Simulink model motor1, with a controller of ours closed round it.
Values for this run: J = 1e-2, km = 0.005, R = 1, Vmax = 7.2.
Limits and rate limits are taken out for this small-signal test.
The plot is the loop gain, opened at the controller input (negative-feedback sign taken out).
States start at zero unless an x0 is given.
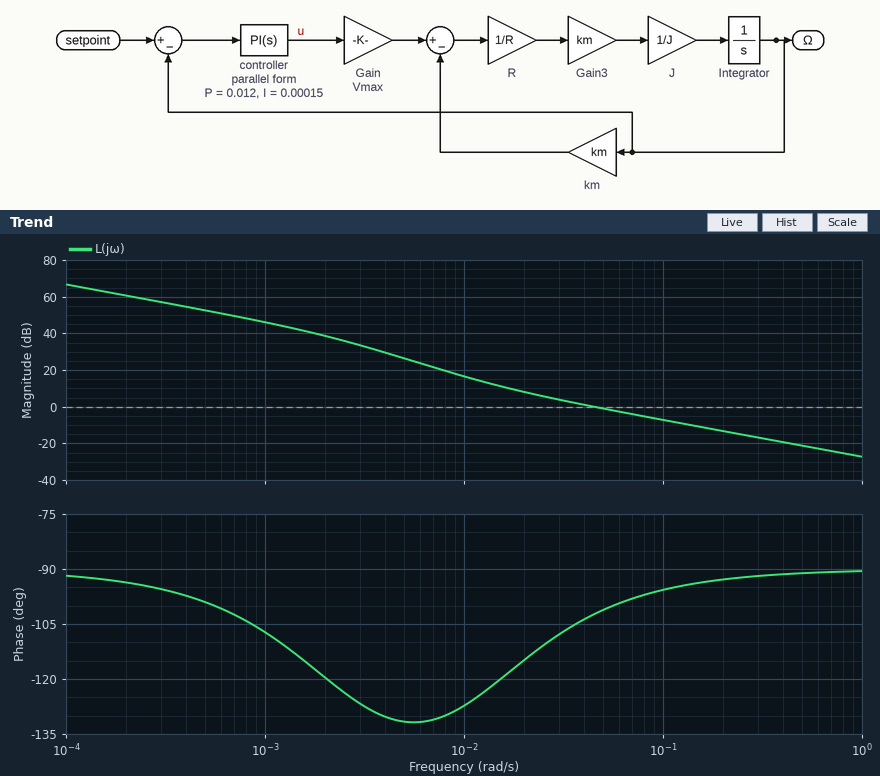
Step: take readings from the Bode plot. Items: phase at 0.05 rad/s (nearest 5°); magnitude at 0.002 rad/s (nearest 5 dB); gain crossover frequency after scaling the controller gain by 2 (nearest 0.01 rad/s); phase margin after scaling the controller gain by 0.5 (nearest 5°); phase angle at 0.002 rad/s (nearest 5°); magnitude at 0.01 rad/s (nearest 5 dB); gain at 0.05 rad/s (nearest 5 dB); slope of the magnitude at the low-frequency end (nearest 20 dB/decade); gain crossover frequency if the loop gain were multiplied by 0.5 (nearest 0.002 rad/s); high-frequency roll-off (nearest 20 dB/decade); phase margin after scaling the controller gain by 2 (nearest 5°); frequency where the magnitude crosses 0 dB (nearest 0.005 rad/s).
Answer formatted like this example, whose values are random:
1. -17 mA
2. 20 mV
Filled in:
1. -100°
2. 40 dB
3. 0.09 rad/s
4. 70°
5. -120°
6. 15 dB
7. 0 dB
8. -20 dB/decade
9. 0.024 rad/s
10. -20 dB/decade
11. 85°
12. 0.045 rad/s
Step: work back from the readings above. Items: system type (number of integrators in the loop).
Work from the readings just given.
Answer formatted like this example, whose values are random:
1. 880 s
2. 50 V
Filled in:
1. 1
